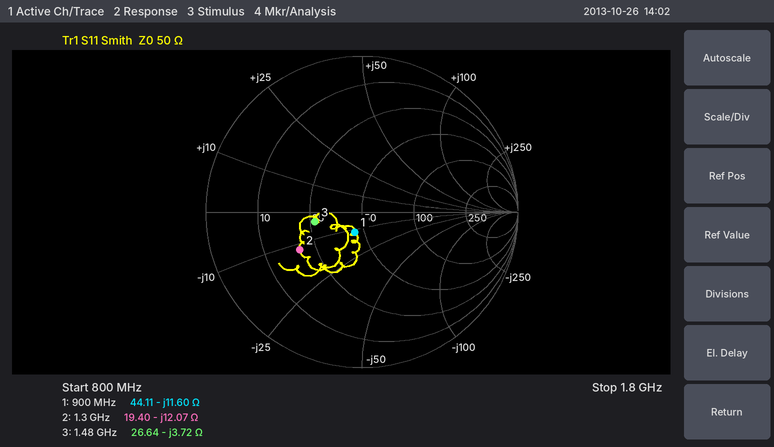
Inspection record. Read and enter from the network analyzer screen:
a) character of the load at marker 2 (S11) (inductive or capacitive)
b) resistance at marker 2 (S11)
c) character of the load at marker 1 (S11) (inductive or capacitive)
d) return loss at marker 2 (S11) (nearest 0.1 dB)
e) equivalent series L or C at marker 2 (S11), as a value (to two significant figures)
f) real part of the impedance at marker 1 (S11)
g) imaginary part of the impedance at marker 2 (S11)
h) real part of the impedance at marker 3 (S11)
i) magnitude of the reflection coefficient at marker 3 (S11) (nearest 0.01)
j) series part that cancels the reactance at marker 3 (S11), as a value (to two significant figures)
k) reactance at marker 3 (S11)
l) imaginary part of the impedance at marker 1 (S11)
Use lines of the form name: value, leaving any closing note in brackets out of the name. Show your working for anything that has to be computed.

character of the load at marker 2 (S11): capacitive
resistance at marker 2: 19.40 Ω
character of the load at marker 1 (S11): capacitive
return loss at marker 2 (S11): 6.6 dB
equivalent series L or C at marker 2 (S11), as a value: C = 1/(2π × 1.3 GHz × 12.07 Ω) ≈ 10 pF
real part of the impedance at marker 1: 44.11 Ω
imaginary part of the impedance at marker 2: -12.07 Ω
real part of the impedance at marker 3: 26.64 Ω
magnitude of the reflection coefficient at marker 3 (S11): 0.31
series part that cancels the reactance at marker 3 (S11), as a value: L = 3.72 Ω/(2π × 1.48 GHz) ≈ 400 pH
reactance at marker 3: -3.72 Ω
imaginary part of the impedance at marker 1: -11.60 Ω
